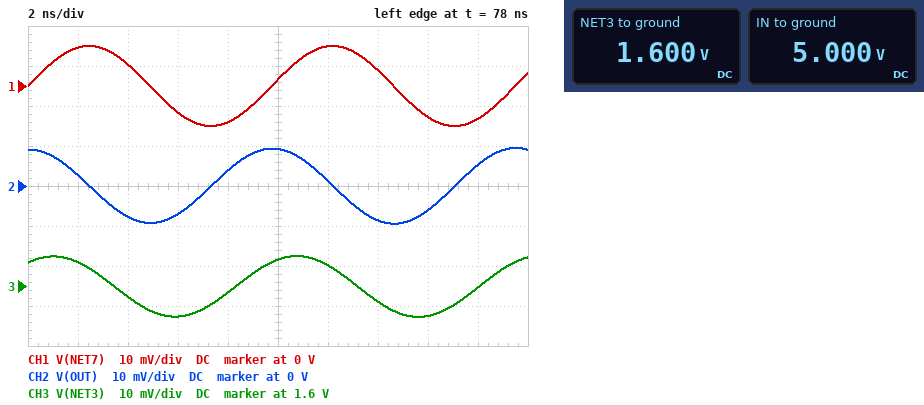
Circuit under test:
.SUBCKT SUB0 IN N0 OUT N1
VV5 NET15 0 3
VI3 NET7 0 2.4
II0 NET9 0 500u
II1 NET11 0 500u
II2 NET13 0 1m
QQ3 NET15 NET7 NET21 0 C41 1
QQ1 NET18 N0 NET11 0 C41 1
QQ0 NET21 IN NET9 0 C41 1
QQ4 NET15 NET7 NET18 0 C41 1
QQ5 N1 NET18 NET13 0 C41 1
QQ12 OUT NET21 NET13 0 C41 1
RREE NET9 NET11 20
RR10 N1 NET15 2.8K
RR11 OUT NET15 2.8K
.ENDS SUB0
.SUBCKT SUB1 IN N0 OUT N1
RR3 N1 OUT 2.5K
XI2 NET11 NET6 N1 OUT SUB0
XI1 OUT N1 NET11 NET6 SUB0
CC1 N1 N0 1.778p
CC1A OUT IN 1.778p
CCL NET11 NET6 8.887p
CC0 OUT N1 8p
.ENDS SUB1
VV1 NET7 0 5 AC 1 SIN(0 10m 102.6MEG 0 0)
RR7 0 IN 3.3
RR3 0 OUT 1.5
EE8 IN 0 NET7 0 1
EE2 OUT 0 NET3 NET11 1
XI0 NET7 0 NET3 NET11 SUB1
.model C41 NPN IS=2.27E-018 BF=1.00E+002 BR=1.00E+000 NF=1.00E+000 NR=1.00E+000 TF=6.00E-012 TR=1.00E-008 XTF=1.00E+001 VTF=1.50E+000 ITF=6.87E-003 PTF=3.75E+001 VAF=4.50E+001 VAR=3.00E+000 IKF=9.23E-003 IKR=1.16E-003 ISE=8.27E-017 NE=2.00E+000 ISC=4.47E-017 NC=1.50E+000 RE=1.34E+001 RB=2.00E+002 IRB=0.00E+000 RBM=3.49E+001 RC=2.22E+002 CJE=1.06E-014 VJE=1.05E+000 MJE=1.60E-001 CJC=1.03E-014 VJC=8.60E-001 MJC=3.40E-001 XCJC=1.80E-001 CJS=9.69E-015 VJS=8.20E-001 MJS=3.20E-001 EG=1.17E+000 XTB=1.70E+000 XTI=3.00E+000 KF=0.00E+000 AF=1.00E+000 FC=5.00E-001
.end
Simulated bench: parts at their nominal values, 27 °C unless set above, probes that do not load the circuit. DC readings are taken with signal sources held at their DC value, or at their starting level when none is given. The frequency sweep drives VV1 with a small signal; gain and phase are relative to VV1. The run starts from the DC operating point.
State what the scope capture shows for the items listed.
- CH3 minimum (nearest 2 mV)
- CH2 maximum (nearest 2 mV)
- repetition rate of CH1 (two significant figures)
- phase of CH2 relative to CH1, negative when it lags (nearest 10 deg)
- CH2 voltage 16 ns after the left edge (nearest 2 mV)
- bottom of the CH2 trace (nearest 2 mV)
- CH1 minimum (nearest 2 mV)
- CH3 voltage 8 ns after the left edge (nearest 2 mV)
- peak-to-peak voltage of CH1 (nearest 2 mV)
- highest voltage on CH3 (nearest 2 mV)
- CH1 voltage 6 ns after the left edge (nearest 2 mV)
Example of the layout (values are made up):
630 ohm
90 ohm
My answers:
1.592 V
10 mV
100 MHz
90 deg
-6 mV
-10 mV
-10 mV
1.598 V
20 mV
1.608 V
-6 mV
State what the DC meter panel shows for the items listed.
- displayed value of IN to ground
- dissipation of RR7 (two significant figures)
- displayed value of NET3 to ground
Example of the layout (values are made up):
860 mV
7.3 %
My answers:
5.000 V
7.6 W
1.600 V
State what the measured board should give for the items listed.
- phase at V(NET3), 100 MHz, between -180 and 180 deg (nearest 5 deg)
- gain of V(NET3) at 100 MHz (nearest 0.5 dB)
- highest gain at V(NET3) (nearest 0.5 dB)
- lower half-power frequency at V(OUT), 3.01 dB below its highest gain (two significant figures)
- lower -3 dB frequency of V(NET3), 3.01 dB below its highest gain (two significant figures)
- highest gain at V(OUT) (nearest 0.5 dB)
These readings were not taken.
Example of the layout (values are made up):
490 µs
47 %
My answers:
65 deg
-4.5 dB
-1.5 dB
98 MHz
100 MHz
0 dB
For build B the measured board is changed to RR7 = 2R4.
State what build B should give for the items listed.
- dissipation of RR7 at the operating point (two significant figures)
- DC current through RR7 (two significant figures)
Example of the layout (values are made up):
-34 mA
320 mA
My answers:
10 W
2.1 A
